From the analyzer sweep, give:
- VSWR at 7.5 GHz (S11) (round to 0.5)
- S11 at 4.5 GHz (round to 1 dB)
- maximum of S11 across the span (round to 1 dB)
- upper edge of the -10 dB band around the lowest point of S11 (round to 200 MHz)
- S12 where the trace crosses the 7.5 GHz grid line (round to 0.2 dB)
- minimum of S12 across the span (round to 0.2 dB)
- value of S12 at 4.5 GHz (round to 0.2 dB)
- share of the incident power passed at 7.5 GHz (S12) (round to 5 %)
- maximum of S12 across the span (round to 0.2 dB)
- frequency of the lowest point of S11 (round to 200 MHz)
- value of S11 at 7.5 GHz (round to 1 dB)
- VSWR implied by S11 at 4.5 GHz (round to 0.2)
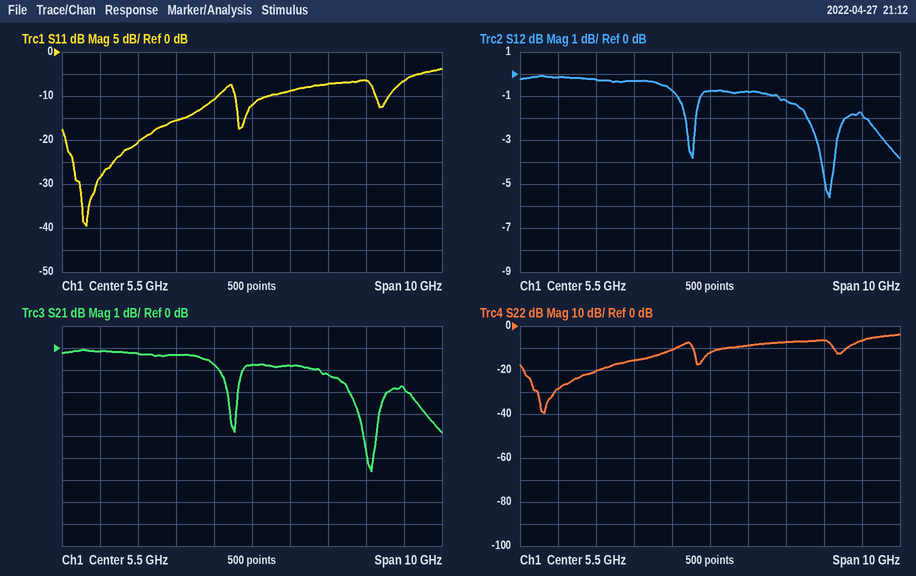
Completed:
2.5
-11 dB
-4 dB
4.6 GHz
-1.2 dB
-5.6 dB
-0.8 dB
75 %
0.0 dB
1.2 GHz
-7 dB
1.8
